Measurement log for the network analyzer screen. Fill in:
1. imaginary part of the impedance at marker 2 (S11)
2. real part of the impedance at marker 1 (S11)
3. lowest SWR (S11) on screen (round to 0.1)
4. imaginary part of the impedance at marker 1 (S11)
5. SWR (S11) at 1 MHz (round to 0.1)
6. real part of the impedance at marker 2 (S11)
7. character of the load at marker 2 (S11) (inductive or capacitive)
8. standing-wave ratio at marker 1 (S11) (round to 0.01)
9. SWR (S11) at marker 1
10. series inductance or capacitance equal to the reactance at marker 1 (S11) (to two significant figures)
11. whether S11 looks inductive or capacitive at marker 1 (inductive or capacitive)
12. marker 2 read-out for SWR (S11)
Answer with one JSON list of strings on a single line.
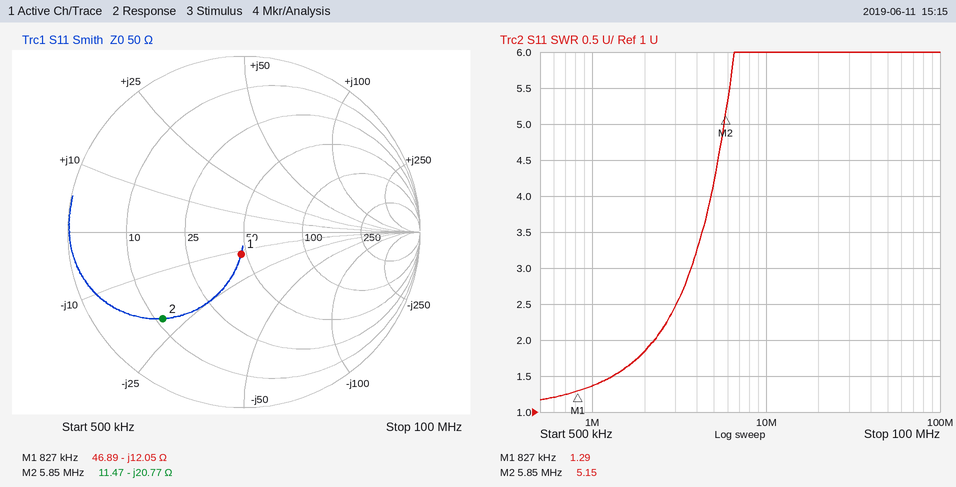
["-20.77 Ω", "46.89 Ω", "1.2", "-12.05 Ω", "1.4", "11.47 Ω", "capacitive", "1.29", "1.29", "16 nF", "capacitive", "5.15"]
